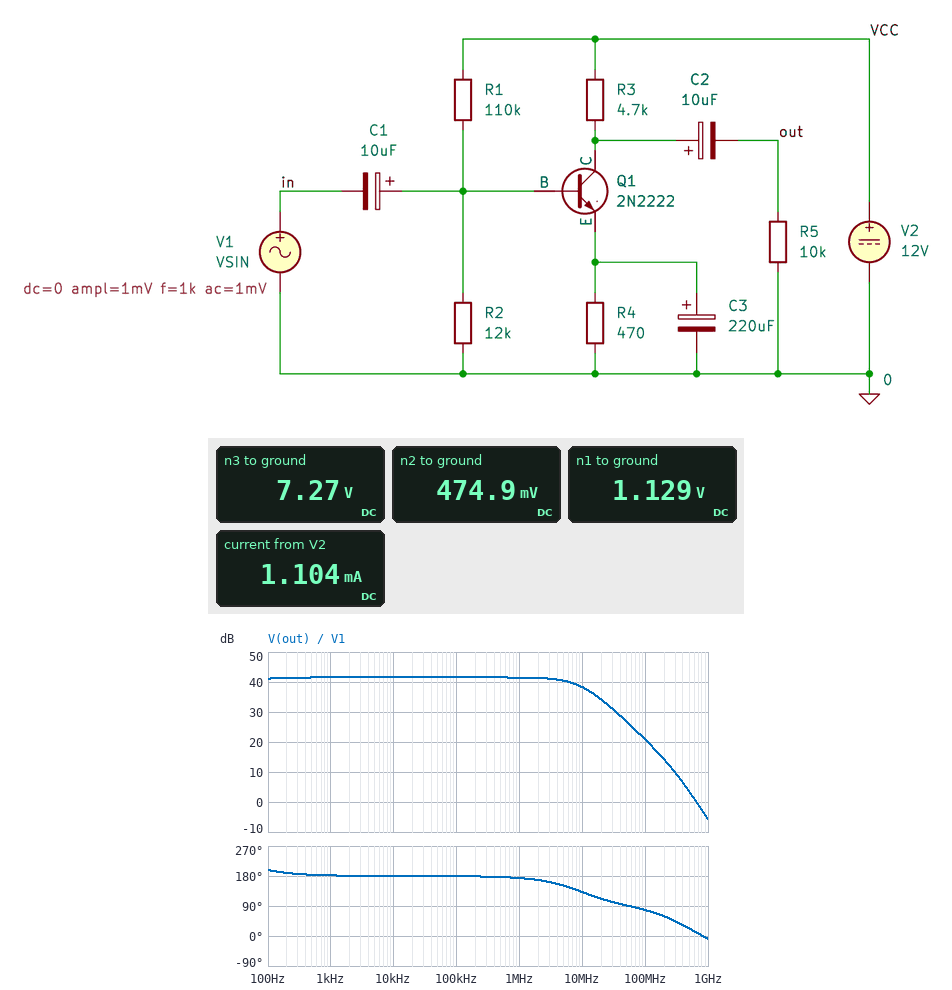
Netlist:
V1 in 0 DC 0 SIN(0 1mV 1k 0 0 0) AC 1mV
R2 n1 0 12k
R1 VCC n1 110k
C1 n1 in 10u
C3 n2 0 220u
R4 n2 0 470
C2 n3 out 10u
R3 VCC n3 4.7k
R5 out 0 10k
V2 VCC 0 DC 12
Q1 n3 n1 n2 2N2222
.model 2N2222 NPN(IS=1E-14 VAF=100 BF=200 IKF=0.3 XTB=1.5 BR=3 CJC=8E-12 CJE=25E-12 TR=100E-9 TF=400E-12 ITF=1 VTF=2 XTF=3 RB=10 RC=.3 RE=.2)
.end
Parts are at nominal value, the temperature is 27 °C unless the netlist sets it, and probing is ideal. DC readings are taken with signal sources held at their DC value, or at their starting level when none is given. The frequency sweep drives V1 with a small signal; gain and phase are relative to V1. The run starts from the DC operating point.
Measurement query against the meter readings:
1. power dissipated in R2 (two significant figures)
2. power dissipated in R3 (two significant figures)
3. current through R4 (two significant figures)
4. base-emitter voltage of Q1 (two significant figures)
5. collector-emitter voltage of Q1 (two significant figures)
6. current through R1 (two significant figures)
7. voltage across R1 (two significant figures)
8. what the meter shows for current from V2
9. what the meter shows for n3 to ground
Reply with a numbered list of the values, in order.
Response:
1. 110 µW
2. 4.8 mW
3. 1.0 mA
4. 650 mV
5. 6.8 V
6. 99 µA
7. 11 V
8. 1.104 mA
9. 7.27 V
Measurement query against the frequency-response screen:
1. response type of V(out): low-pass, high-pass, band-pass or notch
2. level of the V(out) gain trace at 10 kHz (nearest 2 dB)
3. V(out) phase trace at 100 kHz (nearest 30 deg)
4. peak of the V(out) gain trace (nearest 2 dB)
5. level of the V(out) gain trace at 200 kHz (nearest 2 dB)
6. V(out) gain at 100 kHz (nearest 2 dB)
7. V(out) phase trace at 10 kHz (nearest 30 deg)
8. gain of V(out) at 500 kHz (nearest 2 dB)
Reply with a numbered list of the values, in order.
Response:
1. low-pass
2. 42 dB
3. 180 deg
4. 42 dB
5. 42 dB
6. 42 dB
7. 180 deg
8. 42 dB
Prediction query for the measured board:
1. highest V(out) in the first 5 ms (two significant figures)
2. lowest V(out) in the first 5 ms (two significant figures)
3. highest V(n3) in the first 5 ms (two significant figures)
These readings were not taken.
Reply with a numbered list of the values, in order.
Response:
1. 120 mV
2. -120 mV
3. 7.4 V
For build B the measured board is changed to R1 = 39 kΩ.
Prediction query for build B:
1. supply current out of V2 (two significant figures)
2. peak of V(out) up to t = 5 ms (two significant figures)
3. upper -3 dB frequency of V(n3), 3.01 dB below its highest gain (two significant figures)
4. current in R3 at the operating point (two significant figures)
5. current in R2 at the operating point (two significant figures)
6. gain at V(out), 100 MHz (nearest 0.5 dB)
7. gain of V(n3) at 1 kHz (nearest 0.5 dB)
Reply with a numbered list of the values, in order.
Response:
1. 2.6 mA
2. 5.3 mV
3. 1.3 MHz
4. 2.3 mA
5. 150 µA
6. -6.5 dB
7. 13.0 dB
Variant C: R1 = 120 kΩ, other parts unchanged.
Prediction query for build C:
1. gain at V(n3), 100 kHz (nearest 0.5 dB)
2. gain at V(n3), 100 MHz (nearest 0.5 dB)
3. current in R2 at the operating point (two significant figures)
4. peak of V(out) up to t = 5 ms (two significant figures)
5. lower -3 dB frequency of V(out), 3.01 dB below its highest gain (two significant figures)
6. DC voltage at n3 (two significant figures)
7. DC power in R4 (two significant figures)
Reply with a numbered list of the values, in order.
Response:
1. 40.0 dB
2. 20.0 dB
3. 87 µA
4. 100 mV
5. 27 Hz
6. 8.0 V
7. 340 µW
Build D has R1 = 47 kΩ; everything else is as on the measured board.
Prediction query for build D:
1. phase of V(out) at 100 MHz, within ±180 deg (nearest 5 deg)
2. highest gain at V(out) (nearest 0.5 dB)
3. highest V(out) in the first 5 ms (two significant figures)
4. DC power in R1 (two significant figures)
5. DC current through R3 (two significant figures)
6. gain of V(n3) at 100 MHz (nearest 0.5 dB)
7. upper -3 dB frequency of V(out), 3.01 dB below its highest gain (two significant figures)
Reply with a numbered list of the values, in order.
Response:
1. 0 deg
2. 18.0 dB
3. 10 mV
4. 2.2 mW
5. 2.3 mA
6. -6.0 dB
7. 1.3 MHz
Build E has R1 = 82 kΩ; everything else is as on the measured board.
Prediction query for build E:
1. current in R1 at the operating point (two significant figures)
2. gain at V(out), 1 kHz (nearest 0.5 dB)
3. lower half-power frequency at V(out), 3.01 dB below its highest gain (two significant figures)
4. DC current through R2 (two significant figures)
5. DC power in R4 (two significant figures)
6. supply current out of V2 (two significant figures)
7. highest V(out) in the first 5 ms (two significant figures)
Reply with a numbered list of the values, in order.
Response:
1. 130 µA
2. 45.5 dB
3. 50 Hz
4. 120 µA
5. 1.3 mW
6. 1.8 mA
7. 190 mV
